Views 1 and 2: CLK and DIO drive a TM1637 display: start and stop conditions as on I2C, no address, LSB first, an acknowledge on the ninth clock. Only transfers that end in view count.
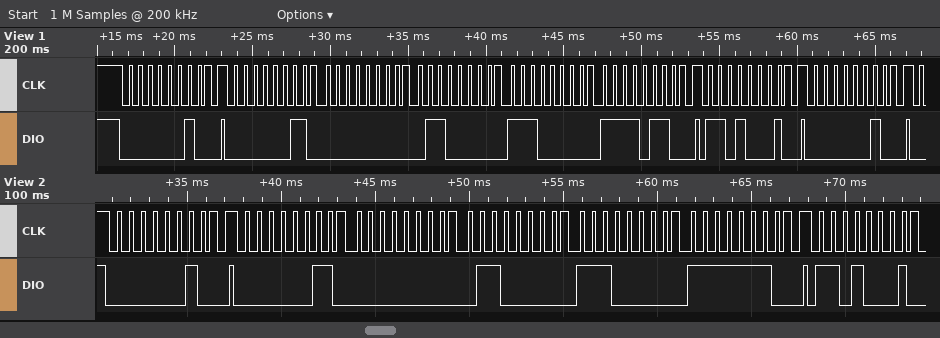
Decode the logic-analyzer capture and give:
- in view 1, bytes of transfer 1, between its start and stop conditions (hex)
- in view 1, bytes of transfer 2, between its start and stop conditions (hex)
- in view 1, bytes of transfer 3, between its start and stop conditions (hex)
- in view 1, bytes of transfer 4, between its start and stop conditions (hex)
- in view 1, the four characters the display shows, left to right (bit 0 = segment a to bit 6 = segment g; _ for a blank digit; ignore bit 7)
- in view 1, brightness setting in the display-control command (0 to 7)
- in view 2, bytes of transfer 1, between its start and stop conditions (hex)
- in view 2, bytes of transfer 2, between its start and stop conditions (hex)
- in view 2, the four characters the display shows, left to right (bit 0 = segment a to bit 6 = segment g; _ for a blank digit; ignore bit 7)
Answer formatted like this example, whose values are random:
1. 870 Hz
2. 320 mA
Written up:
1. 40
2. C0 00 06 07 6F
3. 8B
4. 40
5. _179
6. 3
7. 40
8. C0 00 06 07 7F
9. _178
